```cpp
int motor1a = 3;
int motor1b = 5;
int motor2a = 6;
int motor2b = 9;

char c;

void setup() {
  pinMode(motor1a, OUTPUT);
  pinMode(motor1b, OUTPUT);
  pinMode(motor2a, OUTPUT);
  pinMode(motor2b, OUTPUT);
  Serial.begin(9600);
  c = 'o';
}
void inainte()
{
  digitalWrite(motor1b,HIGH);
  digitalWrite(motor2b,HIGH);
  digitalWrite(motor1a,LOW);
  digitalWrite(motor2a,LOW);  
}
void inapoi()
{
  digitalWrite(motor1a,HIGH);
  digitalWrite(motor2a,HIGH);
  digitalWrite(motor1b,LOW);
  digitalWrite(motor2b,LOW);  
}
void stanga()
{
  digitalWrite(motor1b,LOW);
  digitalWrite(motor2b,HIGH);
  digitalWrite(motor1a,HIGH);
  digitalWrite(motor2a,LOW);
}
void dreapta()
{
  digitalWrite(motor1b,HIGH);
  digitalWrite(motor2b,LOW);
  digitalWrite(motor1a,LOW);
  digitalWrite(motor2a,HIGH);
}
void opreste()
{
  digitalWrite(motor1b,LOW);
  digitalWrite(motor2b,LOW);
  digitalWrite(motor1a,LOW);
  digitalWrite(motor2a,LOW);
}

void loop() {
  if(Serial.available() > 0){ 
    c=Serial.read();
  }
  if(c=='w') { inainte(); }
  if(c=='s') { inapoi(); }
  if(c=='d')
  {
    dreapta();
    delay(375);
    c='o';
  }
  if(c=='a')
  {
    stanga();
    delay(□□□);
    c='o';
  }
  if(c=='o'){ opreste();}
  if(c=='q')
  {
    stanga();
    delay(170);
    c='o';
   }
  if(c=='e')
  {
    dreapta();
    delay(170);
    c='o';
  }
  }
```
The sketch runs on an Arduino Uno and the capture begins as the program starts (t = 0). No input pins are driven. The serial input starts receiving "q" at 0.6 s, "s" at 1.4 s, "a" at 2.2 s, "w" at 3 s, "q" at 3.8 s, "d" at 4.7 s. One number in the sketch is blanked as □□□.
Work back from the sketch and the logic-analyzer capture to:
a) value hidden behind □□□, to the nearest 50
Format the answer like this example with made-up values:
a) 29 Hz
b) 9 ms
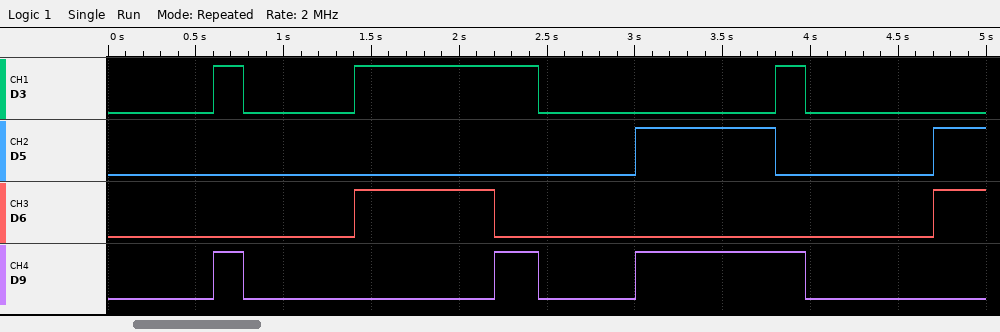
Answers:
a) 250
